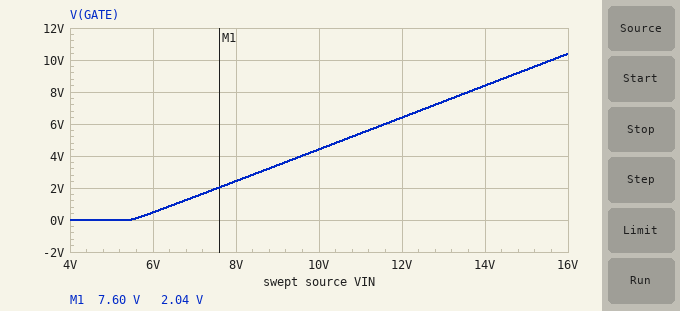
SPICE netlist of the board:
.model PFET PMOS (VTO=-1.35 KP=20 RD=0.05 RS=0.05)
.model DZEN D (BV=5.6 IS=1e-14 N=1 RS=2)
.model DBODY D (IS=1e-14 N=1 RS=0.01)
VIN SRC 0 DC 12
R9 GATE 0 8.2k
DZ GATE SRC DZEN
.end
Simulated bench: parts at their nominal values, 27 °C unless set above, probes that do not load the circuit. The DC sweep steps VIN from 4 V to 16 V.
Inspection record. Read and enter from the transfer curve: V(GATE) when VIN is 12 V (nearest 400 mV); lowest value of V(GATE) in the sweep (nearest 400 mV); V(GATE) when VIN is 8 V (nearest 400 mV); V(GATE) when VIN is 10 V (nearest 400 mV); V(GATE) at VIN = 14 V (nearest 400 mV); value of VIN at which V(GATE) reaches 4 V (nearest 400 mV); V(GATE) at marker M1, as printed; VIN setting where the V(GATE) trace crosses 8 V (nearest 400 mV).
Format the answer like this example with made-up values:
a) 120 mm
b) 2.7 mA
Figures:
a) 6.4 V
b) 0 V
c) 2.4 V
d) 4.4 V
e) 8.4 V
f) 9.6 V
g) 2.04 V
h) 13.6 V
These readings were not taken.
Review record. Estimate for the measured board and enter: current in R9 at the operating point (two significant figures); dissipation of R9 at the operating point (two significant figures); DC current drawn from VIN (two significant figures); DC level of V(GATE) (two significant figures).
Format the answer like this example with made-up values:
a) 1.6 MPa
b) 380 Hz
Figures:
a) 780 µA
b) 5.0 mW
c) 780 µA
d) 6.4 V
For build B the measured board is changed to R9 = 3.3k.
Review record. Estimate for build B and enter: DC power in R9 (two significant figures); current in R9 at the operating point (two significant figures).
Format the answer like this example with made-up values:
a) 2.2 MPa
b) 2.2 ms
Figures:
a) 12 mW
b) 1.9 mA
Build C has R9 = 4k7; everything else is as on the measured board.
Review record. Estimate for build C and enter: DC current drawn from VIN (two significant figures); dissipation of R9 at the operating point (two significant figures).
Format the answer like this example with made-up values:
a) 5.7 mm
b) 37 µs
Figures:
a) 1.4 mA
b) 8.7 mW
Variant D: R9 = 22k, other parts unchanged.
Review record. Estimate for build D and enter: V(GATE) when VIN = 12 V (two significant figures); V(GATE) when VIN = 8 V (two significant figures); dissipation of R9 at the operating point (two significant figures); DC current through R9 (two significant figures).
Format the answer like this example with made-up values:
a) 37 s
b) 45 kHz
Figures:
a) 6.4 V
b) 2.5 V
c) 1.9 mW
d) 290 µA
